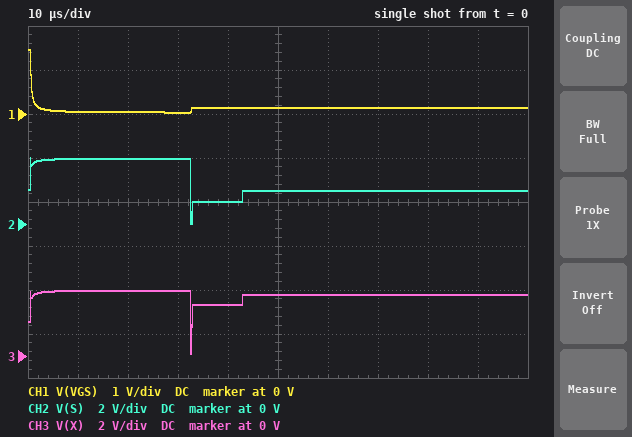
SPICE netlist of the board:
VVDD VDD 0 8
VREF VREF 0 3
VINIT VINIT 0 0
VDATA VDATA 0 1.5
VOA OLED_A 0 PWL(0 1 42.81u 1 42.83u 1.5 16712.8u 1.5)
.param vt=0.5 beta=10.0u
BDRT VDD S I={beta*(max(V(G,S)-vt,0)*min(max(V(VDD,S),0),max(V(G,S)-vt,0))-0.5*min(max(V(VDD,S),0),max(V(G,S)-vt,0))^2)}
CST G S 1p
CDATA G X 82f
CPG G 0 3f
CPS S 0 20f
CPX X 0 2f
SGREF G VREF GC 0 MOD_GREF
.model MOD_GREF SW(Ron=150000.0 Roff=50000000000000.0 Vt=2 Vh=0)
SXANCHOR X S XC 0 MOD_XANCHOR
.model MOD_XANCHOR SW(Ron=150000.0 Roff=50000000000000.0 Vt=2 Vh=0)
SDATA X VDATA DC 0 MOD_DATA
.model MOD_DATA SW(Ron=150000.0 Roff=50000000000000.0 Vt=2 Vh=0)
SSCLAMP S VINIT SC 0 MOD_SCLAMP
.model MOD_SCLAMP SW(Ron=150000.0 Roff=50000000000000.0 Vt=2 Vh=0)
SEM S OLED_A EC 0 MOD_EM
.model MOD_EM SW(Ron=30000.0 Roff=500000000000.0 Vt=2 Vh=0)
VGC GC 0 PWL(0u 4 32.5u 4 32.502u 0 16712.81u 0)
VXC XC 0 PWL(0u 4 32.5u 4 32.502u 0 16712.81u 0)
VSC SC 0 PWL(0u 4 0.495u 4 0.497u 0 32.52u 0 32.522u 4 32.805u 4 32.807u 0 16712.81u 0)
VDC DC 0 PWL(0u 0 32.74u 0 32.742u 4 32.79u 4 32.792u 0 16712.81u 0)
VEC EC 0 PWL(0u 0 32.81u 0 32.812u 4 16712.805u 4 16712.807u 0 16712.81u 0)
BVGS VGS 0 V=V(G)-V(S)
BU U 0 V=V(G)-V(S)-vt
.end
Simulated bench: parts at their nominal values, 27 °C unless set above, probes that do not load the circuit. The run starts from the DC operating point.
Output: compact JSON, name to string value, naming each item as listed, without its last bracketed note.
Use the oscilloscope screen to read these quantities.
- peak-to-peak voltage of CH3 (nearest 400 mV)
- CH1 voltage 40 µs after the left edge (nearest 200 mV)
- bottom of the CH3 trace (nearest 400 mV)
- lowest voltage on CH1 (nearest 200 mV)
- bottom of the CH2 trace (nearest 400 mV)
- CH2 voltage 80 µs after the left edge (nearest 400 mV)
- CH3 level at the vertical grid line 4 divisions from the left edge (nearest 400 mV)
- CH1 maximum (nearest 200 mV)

{"peak-to-peak voltage of CH3": "2.8 V", "CH1 voltage 40 µs after the left edge": "200 mV", "bottom of the CH3 trace": "0 V", "lowest voltage on CH1": "0 V", "bottom of the CH2 trace": "0 V", "CH2 voltage 80 µs after the left edge": "1.6 V", "CH3 level at the vertical grid line 4 divisions from the left edge": "2.4 V", "CH1 maximum": "1.4 V"}
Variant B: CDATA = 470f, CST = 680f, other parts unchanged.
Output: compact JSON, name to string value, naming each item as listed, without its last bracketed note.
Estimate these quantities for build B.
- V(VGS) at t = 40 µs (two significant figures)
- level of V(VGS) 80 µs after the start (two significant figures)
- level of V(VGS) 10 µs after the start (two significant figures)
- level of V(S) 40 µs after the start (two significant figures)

{"V(VGS) at t = 40 µs": "320 mV", "level of V(VGS) 80 µs after the start": "310 mV", "level of V(VGS) 10 µs after the start": "51 mV", "level of V(S) 40 µs after the start": "1.0 V"}
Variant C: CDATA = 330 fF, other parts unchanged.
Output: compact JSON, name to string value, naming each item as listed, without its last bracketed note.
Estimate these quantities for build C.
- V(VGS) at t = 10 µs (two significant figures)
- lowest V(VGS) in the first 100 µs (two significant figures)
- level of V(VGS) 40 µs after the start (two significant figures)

{"V(VGS) at t = 10 µs": "54 mV", "lowest V(VGS) in the first 100 µs": "34 mV", "level of V(VGS) 40 µs after the start": "220 mV"}
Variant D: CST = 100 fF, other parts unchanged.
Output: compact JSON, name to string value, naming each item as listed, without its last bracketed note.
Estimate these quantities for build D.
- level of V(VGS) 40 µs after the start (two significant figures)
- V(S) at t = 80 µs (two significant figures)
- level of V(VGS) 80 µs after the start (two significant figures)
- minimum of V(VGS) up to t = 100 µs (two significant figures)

{"level of V(VGS) 40 µs after the start": "580 mV", "V(S) at t = 80 µs": "1.5 V", "level of V(VGS) 80 µs after the start": "560 mV", "minimum of V(VGS) up to t = 100 µs": "27 mV"}
